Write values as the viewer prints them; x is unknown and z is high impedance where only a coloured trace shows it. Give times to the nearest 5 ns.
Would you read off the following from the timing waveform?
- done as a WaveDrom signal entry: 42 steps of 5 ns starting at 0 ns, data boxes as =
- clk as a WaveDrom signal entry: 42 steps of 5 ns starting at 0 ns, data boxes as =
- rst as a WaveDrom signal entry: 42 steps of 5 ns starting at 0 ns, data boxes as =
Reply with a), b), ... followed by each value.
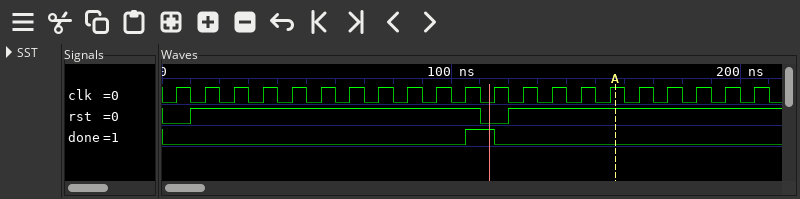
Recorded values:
a) {name: 'done', wave: '0....................1.0..................'}
b) {name: 'clk', wave: '010101010101010101010101010101010101010101'}
c) {name: 'rst', wave: '0.1...................0.1.................'}
